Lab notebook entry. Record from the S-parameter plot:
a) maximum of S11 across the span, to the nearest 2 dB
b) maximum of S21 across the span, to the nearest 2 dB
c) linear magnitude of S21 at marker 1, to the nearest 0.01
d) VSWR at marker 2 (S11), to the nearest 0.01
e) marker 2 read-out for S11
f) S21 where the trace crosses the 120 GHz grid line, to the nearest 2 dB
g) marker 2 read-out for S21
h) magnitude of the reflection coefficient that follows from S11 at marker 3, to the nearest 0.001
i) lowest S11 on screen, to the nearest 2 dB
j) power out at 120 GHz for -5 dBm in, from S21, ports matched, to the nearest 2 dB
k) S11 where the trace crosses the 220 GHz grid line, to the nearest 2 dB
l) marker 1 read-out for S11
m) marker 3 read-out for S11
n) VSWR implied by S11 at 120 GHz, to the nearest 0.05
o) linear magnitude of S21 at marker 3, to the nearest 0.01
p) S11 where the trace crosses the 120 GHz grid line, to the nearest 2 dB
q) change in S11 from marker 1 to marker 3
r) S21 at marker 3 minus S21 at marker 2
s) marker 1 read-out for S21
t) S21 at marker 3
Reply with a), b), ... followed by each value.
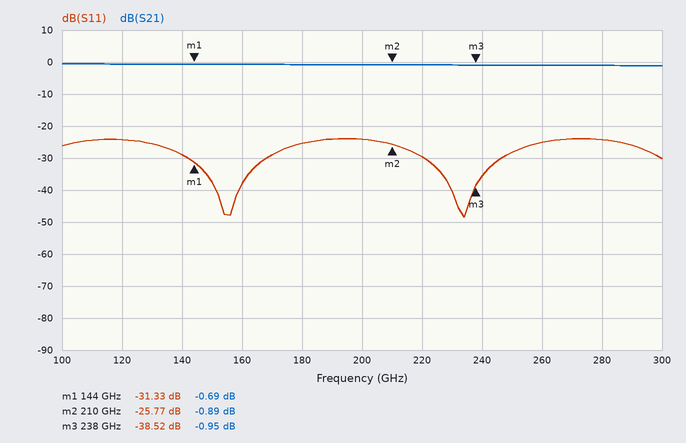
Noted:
a) -24 dB
b) 0 dB
c) 0.92
d) 1.11
e) -25.77 dB
f) 0 dB
g) -0.89 dB
h) 0.012
i) -48 dB
j) -6 dBm
k) -30 dB
l) -31.33 dB
m) -38.52 dB
n) 1.15
o) 0.90
p) -24 dB
q) -7.19 dB
r) -0.06 dB
s) -0.69 dB
t) -0.95 dB
